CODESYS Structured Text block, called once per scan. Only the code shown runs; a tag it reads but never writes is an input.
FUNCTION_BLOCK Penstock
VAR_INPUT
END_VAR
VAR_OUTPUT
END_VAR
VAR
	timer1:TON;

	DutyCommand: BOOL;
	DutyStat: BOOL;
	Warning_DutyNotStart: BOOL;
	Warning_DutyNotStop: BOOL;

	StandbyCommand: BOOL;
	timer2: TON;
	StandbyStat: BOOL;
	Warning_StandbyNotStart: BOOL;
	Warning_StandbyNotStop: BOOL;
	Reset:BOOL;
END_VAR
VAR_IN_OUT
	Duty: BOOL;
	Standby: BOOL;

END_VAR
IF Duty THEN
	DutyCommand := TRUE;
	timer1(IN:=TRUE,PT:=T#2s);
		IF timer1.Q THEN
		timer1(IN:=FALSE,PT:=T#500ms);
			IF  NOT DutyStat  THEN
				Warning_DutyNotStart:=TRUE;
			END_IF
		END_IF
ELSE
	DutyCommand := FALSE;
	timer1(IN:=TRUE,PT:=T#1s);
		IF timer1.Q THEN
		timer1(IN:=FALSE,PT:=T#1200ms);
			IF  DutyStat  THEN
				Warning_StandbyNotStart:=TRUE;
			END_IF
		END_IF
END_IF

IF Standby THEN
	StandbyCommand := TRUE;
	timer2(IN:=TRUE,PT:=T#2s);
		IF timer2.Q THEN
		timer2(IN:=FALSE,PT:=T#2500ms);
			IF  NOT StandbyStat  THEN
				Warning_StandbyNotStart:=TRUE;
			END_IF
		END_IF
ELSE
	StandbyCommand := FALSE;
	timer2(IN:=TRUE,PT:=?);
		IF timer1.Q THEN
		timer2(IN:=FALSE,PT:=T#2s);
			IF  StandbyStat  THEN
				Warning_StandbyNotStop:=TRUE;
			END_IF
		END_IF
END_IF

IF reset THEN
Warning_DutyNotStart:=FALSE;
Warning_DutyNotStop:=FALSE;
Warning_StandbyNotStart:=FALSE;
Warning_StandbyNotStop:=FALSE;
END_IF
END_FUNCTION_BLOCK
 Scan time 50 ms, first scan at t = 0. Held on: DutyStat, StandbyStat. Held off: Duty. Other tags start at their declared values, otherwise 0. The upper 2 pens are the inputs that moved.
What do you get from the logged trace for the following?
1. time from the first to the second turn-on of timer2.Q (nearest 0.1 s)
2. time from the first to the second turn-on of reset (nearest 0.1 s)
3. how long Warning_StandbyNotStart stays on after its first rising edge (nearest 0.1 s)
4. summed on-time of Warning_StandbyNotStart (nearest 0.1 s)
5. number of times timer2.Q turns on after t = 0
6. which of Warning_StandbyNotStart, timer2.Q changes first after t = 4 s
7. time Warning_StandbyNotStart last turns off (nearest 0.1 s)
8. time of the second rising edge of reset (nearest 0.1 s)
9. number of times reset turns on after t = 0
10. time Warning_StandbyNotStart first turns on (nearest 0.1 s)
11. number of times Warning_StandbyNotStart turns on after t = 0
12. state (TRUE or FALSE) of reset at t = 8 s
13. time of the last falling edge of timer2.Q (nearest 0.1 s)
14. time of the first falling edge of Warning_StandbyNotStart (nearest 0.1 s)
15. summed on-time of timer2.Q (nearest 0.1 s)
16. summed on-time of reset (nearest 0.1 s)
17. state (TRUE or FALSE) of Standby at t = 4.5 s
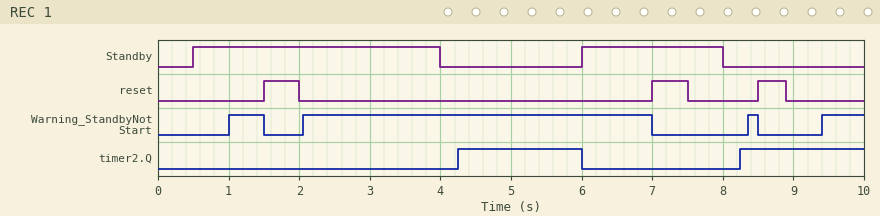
4.0 s
5.5 s
0.5 s
6.2 s
2
timer2.Q
8.5 s
7.0 s
3
1.0 s
4
FALSE
6.0 s
1.5 s
3.5 s
1.4 s
FALSE
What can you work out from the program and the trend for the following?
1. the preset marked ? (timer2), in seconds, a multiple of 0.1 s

2.2 s
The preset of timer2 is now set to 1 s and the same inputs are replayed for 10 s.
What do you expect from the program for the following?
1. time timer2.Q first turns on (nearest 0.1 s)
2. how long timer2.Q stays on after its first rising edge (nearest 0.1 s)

4.0 s
2.0 s
